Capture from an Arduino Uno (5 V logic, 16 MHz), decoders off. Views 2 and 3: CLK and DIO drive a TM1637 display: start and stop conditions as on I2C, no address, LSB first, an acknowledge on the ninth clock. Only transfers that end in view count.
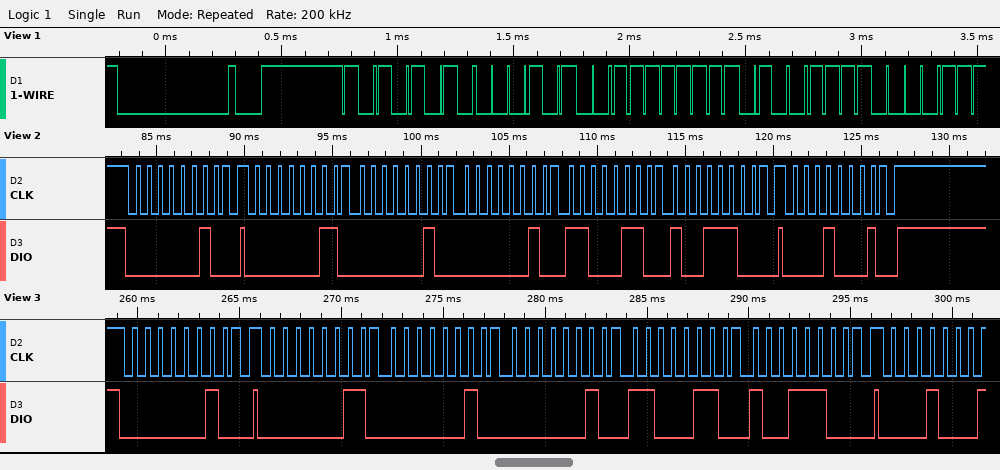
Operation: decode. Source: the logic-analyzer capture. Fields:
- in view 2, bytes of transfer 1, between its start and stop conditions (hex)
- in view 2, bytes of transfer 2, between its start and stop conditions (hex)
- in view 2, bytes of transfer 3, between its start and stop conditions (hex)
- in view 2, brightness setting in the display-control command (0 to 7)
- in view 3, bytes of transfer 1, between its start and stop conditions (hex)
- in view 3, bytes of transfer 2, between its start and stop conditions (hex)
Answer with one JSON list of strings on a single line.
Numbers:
["40", "C0 40 40 63 39", "88", "0", "40", "C0 40 40 63 39"]
